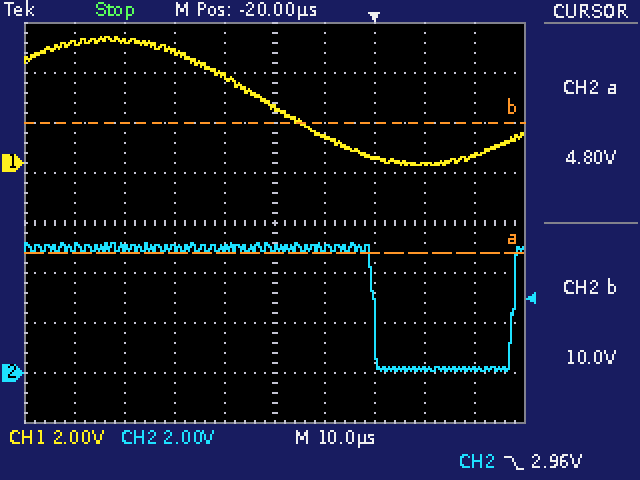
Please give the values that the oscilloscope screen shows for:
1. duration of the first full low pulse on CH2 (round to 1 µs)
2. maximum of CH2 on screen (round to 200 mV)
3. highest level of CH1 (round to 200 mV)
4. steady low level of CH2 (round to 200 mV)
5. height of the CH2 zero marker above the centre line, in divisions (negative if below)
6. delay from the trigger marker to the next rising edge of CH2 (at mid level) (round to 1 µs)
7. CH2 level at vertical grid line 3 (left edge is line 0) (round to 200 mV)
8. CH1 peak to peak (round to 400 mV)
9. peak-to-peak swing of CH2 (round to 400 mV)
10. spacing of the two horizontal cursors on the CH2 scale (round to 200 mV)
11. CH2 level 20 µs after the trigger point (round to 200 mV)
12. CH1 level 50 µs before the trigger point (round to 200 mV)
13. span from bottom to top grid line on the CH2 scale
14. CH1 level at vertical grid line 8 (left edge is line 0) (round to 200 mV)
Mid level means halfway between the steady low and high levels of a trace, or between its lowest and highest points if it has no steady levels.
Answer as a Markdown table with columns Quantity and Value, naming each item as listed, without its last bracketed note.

| Quantity | Value |
|---|---|
| duration of the first full low pulse on CH2 | 28 µs |
| maximum of CH2 on screen | 5.2 V |
| highest level of CH1 | 5.0 V |
| steady low level of CH2 | 200 mV |
| height of the CH2 zero marker above the centre line, in divisions | -3.0 div |
| delay from the trigger marker to the next rising edge of CH2 (at mid level) | 28 µs |
| CH2 level at vertical grid line 3 (left edge is line 0) | 5.0 V |
| CH1 peak to peak | 5.2 V |
| peak-to-peak swing of CH2 | 5.2 V |
| spacing of the two horizontal cursors on the CH2 scale | 5.2 V |
| CH2 level 20 µs after the trigger point | 200 mV |
| CH1 level 50 µs before the trigger point | 4.8 V |
| span from bottom to top grid line on the CH2 scale | 16 V |
| CH1 level at vertical grid line 8 (left edge is line 0) | 0.0 V |
